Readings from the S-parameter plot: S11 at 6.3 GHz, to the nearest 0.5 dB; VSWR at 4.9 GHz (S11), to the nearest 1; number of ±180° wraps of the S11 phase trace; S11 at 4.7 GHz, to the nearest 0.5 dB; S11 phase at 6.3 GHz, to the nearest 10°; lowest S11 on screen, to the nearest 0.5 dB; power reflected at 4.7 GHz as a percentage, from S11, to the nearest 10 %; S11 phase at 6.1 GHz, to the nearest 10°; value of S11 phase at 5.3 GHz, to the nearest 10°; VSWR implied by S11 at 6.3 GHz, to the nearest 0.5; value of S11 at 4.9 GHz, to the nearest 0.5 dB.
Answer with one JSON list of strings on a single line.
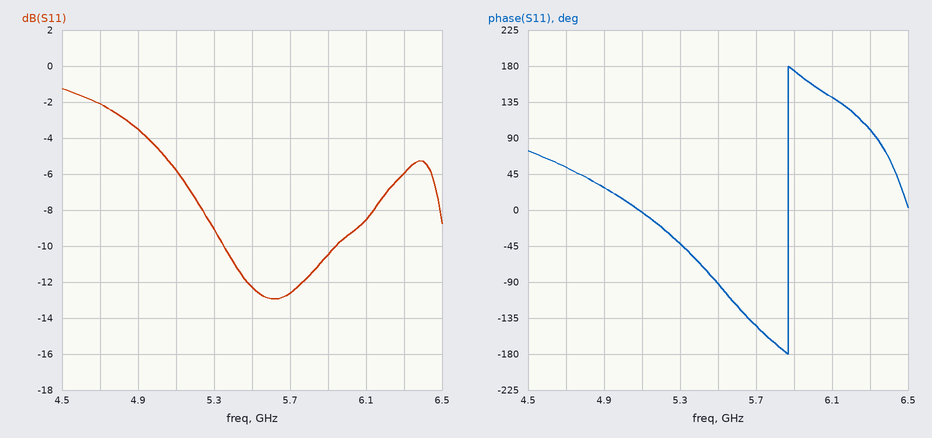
["-6.0 dB", "5", "1", "-2.0 dB", "100°", "-13.0 dB", "60 %", "140°", "-40°", "3.0", "-3.5 dB"]
